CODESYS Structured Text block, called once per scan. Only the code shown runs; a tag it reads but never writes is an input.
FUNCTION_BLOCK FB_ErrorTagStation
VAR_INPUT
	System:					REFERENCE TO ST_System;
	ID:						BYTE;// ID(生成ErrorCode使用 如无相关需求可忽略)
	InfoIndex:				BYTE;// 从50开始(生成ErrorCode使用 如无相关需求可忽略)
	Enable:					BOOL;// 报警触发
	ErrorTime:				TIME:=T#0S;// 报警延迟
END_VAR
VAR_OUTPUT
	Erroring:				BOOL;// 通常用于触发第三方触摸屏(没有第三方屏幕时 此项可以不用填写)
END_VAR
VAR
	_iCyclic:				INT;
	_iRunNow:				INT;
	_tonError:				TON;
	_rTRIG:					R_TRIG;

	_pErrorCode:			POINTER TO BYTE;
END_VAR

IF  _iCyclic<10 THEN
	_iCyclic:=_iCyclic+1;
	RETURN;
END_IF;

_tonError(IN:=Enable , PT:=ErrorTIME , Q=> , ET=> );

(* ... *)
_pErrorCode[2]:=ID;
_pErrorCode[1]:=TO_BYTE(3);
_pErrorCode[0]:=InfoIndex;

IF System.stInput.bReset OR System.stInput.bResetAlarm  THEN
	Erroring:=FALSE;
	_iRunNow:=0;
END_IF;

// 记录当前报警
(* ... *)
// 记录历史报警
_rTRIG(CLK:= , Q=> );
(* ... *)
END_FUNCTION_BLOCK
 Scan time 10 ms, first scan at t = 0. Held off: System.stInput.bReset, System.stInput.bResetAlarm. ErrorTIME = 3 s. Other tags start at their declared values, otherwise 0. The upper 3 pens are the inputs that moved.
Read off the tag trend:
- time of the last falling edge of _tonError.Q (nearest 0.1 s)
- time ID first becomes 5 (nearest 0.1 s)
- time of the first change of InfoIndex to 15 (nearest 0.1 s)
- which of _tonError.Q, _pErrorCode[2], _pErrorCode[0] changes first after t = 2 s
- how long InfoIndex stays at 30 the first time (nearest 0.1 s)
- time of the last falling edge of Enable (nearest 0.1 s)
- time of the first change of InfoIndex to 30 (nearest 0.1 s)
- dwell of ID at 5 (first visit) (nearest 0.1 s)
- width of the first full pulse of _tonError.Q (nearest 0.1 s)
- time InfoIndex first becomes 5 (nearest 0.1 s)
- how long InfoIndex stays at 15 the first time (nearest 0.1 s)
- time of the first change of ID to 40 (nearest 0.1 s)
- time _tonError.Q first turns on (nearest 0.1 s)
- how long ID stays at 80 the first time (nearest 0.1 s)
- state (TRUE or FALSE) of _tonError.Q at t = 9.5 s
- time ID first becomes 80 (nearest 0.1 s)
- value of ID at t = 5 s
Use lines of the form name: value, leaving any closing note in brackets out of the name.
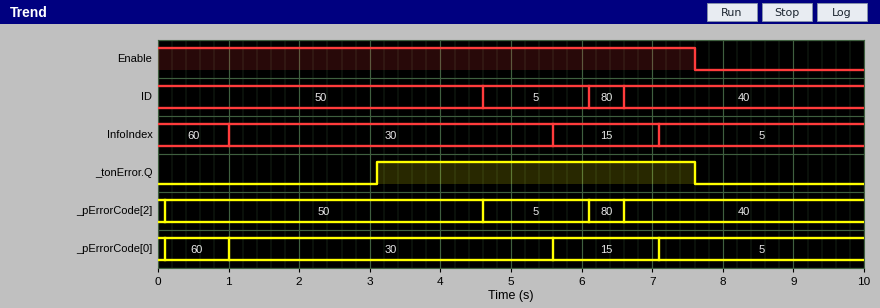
time of the last falling edge of _tonError.Q: 7.6 s
time ID first becomes 5: 4.6 s
time of the first change of InfoIndex to 15: 5.6 s
which of _tonError.Q, _pErrorCode[2], _pErrorCode[0] changes first after t = 2 s: _tonError.Q
how long InfoIndex stays at 30 the first time: 4.6 s
time of the last falling edge of Enable: 7.6 s
time of the first change of InfoIndex to 30: 1.0 s
dwell of ID at 5 (first visit): 1.5 s
width of the first full pulse of _tonError.Q: 4.5 s
time InfoIndex first becomes 5: 7.1 s
how long InfoIndex stays at 15 the first time: 1.5 s
time of the first change of ID to 40: 6.6 s
time _tonError.Q first turns on: 3.1 s
how long ID stays at 80 the first time: 0.5 s
state (TRUE or FALSE) of _tonError.Q at t = 9.5 s: FALSE
time ID first becomes 80: 6.1 s
value of ID at t = 5 s: 5
